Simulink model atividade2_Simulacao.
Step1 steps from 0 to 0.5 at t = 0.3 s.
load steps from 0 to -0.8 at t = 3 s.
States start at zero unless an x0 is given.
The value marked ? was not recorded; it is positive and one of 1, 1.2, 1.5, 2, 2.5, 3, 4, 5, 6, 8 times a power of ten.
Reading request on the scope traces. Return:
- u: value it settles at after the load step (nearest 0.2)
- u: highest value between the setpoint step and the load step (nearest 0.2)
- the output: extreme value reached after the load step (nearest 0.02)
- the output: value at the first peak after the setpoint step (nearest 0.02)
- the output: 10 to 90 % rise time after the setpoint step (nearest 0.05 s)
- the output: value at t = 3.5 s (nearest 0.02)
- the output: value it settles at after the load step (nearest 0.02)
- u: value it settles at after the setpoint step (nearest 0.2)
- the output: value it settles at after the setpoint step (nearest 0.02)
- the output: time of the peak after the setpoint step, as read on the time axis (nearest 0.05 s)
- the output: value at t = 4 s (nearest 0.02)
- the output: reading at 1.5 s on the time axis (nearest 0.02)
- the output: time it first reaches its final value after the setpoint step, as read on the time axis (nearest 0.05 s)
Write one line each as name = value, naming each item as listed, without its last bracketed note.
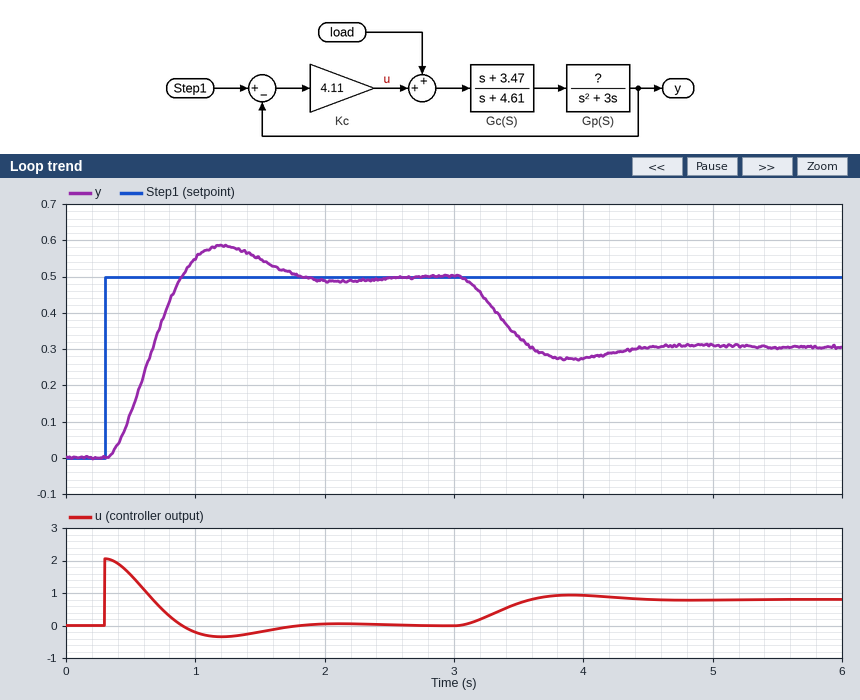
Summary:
u: value it settles at after the load step = 0.8
u: highest value between the setpoint step and the load step = 2.0
the output: extreme value reached after the load step = 0.28
the output: value at the first peak after the setpoint step = 0.58
the output: 10 to 90 % rise time after the setpoint step = 0.40 s
the output: value at t = 3.5 s = 0.34
the output: value it settles at after the load step = 0.30
u: value it settles at after the setpoint step = 0.0
the output: value it settles at after the setpoint step = 0.50
the output: time of the peak after the setpoint step, as read on the time axis = 1.20 s
the output: value at t = 4 s = 0.28
the output: reading at 1.5 s on the time axis = 0.54
the output: time it first reaches its final value after the setpoint step, as read on the time axis = 0.90 s
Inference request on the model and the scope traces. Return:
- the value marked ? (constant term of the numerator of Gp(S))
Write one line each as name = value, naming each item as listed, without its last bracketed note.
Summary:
the value marked ? (constant term of the numerator of Gp(S)) = 4
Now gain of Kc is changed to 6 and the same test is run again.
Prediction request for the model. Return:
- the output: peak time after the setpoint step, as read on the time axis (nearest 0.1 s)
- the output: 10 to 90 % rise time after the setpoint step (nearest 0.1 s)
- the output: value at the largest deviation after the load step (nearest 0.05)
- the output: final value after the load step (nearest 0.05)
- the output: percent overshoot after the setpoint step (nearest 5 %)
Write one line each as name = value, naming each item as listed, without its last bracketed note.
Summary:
the output: peak time after the setpoint step, as read on the time axis = 1.0 s
the output: 10 to 90 % rise time after the setpoint step = 0.3 s
the output: value at the largest deviation after the load step = 0.35
the output: final value after the load step = 0.35
the output: percent overshoot after the setpoint step = 25 %
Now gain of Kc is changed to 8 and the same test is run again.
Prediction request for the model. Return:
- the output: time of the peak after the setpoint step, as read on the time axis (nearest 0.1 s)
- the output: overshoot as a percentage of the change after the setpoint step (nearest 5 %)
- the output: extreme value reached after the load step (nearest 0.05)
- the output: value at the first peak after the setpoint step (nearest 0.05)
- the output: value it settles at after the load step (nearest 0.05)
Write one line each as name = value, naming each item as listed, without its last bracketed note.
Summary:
the output: time of the peak after the setpoint step, as read on the time axis = 0.9 s
the output: overshoot as a percentage of the change after the setpoint step = 30 %
the output: extreme value reached after the load step = 0.35
the output: value at the first peak after the setpoint step = 0.65
the output: value it settles at after the load step = 0.40
